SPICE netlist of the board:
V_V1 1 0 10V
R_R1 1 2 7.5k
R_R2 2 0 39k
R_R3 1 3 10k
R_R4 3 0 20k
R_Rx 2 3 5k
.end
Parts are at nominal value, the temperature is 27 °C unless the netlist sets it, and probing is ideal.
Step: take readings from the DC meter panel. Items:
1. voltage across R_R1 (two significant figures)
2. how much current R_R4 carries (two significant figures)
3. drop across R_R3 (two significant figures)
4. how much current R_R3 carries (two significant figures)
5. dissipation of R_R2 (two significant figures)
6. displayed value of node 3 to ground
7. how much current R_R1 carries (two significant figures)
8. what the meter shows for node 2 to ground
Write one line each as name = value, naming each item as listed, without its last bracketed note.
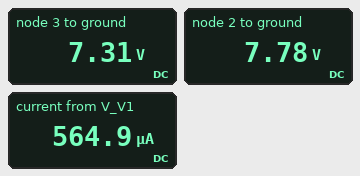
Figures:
voltage across R_R1 = 2.2 V
how much current R_R4 carries = 370 µA
drop across R_R3 = 2.7 V
how much current R_R3 carries = 270 µA
dissipation of R_R2 = 1.6 mW
displayed value of node 3 to ground = 7.31 V
how much current R_R1 carries = 300 µA
what the meter shows for node 2 to ground = 7.78 V
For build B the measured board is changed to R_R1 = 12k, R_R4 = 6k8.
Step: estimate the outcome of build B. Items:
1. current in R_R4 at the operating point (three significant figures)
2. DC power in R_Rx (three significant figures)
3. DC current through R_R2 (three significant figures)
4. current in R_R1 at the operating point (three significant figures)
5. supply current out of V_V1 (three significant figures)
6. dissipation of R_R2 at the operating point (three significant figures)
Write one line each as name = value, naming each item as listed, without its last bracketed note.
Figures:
current in R_R4 at the operating point = 713 µA
DC power in R_Rx = 195 µW
DC current through R_R2 = 150 µA
current in R_R1 at the operating point = 347 µA
supply current out of V_V1 = 862 µA
dissipation of R_R2 at the operating point = 873 µW
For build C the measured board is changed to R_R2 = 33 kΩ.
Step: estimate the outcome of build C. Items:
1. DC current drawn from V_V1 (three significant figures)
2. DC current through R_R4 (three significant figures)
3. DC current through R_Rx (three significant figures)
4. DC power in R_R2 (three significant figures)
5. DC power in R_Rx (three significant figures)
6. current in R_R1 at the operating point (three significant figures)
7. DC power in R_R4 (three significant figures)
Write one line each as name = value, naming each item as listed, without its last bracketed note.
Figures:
DC current drawn from V_V1 = 593 µA
DC current through R_R4 = 361 µA
DC current through R_Rx = 83.3 µA
DC power in R_R2 = 1.77 mW
DC power in R_Rx = 34.7 µW
current in R_R1 at the operating point = 315 µA
DC power in R_R4 = 2.61 mW
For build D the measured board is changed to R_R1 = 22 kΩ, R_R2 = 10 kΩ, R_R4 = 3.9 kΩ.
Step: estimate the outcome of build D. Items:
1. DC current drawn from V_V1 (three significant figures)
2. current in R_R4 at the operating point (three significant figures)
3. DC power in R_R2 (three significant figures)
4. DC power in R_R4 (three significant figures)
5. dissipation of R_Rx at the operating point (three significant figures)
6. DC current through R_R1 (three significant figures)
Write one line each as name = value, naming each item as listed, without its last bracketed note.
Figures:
DC current drawn from V_V1 = 1.03 mA
current in R_R4 at the operating point = 735 µA
DC power in R_R2 = 885 µW
DC power in R_R4 = 2.11 mW
dissipation of R_Rx at the operating point = 2.36 µW
DC current through R_R1 = 319 µA
